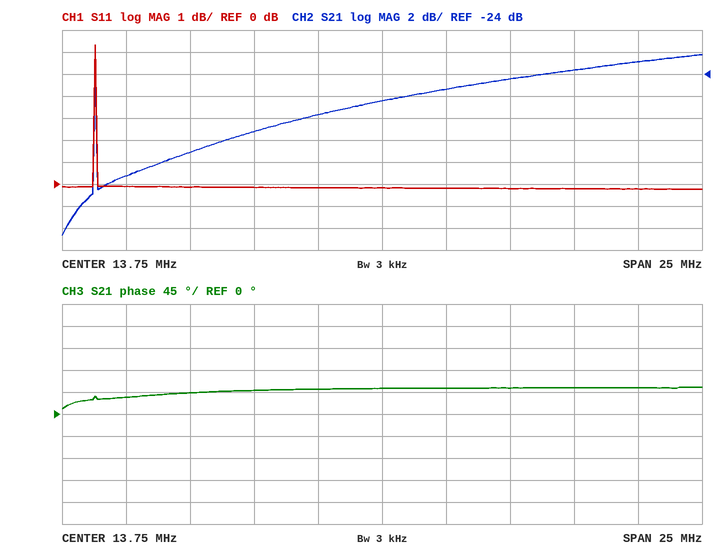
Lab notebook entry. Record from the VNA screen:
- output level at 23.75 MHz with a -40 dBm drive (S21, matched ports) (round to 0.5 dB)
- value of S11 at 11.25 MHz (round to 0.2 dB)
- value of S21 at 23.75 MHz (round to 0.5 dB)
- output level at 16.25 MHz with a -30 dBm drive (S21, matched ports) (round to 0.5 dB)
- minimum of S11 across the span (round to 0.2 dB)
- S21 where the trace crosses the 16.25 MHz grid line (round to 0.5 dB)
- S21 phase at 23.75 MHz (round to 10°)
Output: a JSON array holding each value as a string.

["-63.0 dBm", "-0.2 dB", "-23.0 dB", "-55.5 dBm", "-0.2 dB", "-25.5 dB", "50°"]
